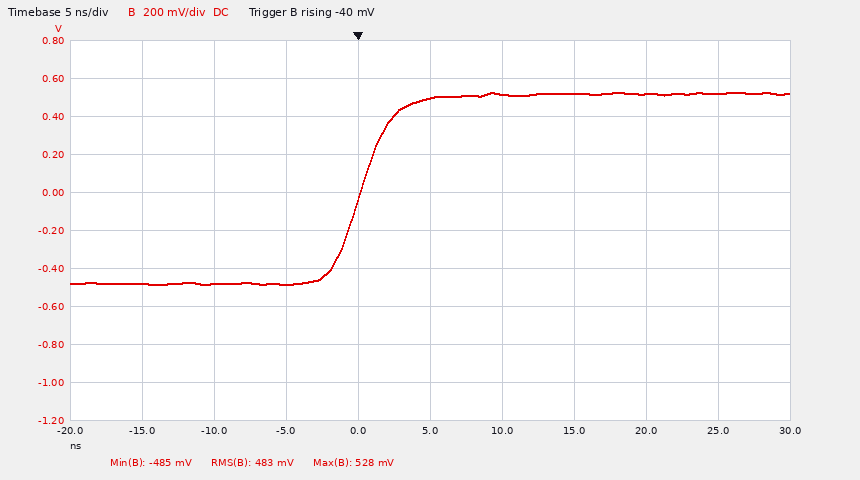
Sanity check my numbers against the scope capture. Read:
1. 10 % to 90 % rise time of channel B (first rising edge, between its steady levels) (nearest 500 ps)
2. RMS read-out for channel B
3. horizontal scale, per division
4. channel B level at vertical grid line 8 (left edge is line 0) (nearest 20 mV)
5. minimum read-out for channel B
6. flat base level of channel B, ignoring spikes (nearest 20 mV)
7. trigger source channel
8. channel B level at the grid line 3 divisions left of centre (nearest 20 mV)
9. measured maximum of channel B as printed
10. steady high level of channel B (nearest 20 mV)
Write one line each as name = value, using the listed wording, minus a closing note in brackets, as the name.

10 % to 90 % rise time of channel B (first rising edge, between its steady levels) = 4.5 ns
RMS read-out for channel B = 483 mV
horizontal scale, per division = 5 ns
channel B level at vertical grid line 8 (left edge is line 0) = 520 mV
minimum read-out for channel B = -485 mV
flat base level of channel B, ignoring spikes = -480 mV
trigger source channel = channel B
channel B level at the grid line 3 divisions left of centre = -480 mV
measured maximum of channel B as printed = 528 mV
steady high level of channel B = 520 mV
